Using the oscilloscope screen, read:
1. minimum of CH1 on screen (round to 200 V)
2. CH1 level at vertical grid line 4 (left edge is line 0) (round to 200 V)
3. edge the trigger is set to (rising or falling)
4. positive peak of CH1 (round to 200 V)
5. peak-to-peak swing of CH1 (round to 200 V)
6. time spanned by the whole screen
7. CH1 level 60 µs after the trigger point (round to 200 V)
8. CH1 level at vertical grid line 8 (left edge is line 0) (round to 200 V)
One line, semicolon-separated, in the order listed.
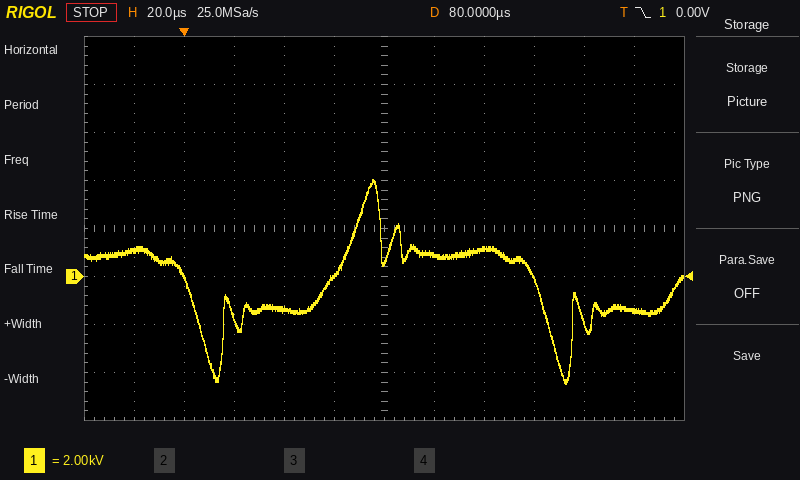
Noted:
-4.4 kV; -1.4 kV; falling; 4.0 kV; 8.4 kV; 240 µs; 0.0 kV; 1.2 kV
